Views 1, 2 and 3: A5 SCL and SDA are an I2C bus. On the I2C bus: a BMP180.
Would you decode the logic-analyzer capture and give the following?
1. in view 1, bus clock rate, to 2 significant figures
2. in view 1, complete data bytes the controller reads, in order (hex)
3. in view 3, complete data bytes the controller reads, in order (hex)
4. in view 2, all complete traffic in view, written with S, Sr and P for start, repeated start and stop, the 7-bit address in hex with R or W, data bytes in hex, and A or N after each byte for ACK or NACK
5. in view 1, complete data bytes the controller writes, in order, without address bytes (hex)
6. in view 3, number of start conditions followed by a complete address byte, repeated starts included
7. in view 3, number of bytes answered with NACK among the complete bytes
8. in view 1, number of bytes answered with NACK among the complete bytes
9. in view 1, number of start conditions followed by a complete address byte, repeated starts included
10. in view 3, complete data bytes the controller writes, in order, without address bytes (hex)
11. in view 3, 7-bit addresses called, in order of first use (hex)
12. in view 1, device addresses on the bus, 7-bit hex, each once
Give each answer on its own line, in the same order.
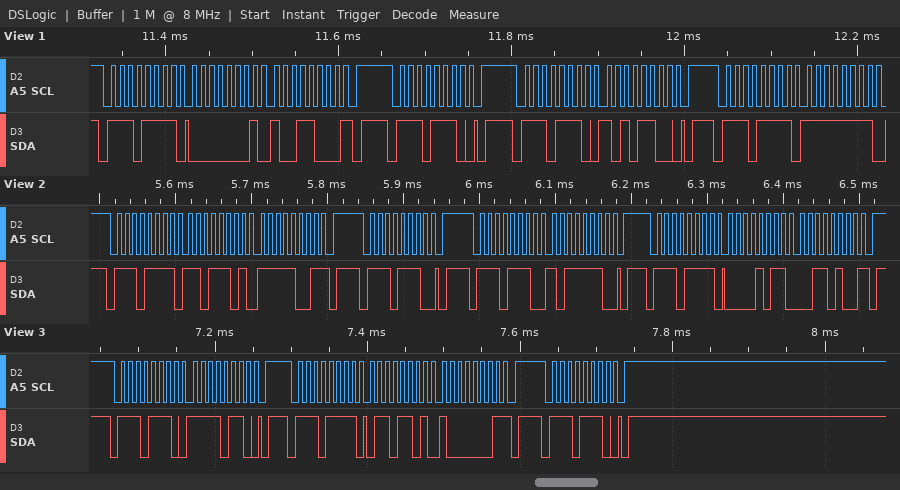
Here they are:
100 kHz
01 98 FF
6D 81
S 77R A DD A F9 N P S 77W A P S 77W A BE A P S 77R A 0B A 34 N P
AC
3
1
1
4
F6
0x77
0x77
